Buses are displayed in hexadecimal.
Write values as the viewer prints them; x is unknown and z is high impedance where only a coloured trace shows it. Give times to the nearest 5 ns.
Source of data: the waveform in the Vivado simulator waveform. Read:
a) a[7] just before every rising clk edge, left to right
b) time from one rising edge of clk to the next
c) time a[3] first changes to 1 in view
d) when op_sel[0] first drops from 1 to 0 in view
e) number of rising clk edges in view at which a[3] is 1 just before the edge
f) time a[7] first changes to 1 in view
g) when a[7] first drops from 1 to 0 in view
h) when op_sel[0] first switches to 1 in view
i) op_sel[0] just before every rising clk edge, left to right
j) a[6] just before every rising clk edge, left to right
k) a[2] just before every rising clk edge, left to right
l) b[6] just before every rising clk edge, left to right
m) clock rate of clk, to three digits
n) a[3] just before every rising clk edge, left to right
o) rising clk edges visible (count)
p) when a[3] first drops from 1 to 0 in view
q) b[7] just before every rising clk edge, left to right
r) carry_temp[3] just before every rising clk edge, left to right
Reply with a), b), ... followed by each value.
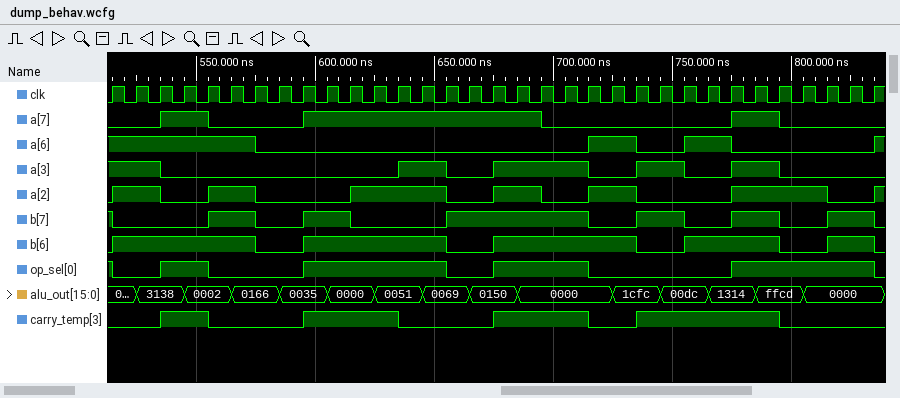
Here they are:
a) 0 0 0 1 1 0 0 0 0 1 1 1 1 1 1 1 1 1 1 0 0 0 0 0 0 0 0 1 1 0 0 0 0
b) 10 ns
c) 635 ns
d) 515 ns
e) 13
f) 535 ns
g) 555 ns
h) 535 ns
i) 1 0 0 1 1 0 0 0 0 1 1 1 1 1 1 0 0 1 1 1 1 0 0 0 0 0 0 1 1 1 1 1 1
j) 1 1 1 1 1 1 1 0 0 0 0 0 0 0 0 0 0 0 0 0 0 1 1 0 0 1 1 0 0 0 0 0 0
k) 0 1 1 0 0 1 1 0 0 0 0 1 1 1 1 0 0 1 1 0 0 1 1 0 0 0 0 1 1 1 1 0 0
l) 0 1 1 1 1 1 1 0 0 1 1 1 1 1 1 0 0 1 1 1 1 1 1 0 0 1 1 1 1 0 0 1 1
m) 100 MHz
n) 1 1 1 0 0 0 0 0 0 0 0 0 0 1 1 0 0 1 1 1 1 0 0 1 1 0 0 1 1 0 0 0 0
o) 33
p) 535 ns
q) 1 0 0 0 0 1 1 0 0 1 1 0 0 0 0 1 1 1 1 1 1 0 0 1 1 0 0 1 1 0 0 1 1
r) 0 0 0 1 1 0 0 0 0 1 1 1 1 0 0 0 0 1 1 1 1 0 0 1 1 1 1 1 1 0 0 0 0
